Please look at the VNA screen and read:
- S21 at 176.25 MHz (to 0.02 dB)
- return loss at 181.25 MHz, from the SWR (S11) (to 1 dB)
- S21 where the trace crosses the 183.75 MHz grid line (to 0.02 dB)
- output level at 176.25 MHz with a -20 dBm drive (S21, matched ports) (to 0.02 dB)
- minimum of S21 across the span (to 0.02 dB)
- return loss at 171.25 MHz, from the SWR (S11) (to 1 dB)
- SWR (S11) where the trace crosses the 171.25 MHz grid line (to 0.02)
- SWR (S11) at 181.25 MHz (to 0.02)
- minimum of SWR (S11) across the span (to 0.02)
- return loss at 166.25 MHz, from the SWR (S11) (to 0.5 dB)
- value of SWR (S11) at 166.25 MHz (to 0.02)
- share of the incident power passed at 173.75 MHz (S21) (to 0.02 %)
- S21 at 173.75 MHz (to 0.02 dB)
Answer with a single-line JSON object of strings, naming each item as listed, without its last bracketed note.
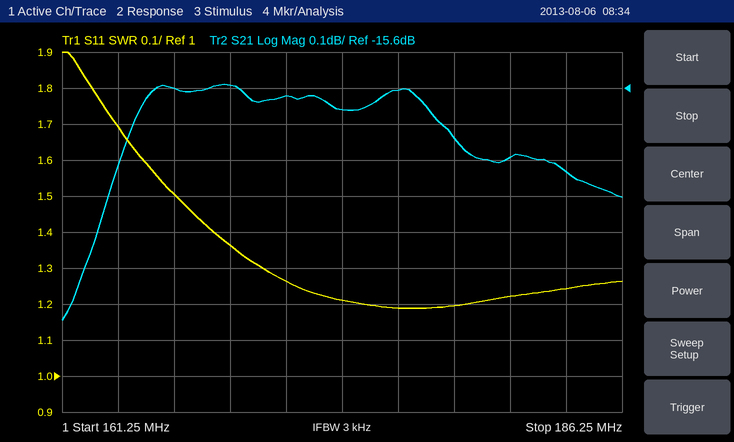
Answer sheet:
{"S21 at 176.25 MHz": "-15.60 dB", "return loss at 181.25 MHz, from the SWR (S11)": "20 dB", "S21 where the trace crosses the 183.75 MHz grid line": "-15.84 dB", "output level at 176.25 MHz with a -20 dBm drive (S21, matched ports)": "-35.60 dBm", "minimum of S21 across the span": "-16.24 dB", "return loss at 171.25 MHz, from the SWR (S11)": "19 dB", "SWR (S11) where the trace crosses the 171.25 MHz grid line": "1.26", "SWR (S11) at 181.25 MHz": "1.22", "minimum of SWR (S11) across the span": "1.18", "return loss at 166.25 MHz, from the SWR (S11)": "14.0 dB", "value of SWR (S11) at 166.25 MHz": "1.50", "share of the incident power passed at 173.75 MHz (S21)": "2.72 %", "S21 at 173.75 MHz": "-15.66 dB"}
